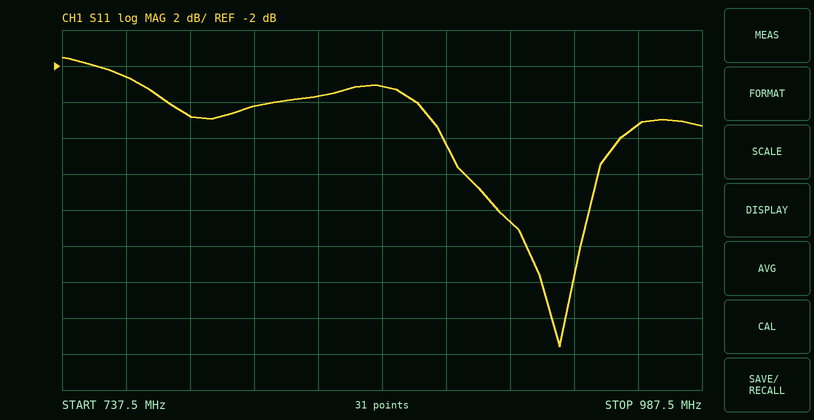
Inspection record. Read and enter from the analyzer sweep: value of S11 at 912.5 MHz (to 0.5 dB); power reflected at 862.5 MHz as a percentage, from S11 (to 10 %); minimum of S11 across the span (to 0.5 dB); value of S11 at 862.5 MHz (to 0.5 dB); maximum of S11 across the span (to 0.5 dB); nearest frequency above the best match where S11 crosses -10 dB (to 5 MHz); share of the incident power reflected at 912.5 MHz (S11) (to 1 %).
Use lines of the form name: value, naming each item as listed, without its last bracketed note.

value of S11 at 912.5 MHz: -10.5 dB
power reflected at 862.5 MHz as a percentage, from S11: 50 %
minimum of S11 across the span: -17.5 dB
value of S11 at 862.5 MHz: -3.0 dB
maximum of S11 across the span: -1.5 dB
nearest frequency above the best match where S11 crosses -10 dB: 945 MHz
share of the incident power reflected at 912.5 MHz (S11): 9 %
